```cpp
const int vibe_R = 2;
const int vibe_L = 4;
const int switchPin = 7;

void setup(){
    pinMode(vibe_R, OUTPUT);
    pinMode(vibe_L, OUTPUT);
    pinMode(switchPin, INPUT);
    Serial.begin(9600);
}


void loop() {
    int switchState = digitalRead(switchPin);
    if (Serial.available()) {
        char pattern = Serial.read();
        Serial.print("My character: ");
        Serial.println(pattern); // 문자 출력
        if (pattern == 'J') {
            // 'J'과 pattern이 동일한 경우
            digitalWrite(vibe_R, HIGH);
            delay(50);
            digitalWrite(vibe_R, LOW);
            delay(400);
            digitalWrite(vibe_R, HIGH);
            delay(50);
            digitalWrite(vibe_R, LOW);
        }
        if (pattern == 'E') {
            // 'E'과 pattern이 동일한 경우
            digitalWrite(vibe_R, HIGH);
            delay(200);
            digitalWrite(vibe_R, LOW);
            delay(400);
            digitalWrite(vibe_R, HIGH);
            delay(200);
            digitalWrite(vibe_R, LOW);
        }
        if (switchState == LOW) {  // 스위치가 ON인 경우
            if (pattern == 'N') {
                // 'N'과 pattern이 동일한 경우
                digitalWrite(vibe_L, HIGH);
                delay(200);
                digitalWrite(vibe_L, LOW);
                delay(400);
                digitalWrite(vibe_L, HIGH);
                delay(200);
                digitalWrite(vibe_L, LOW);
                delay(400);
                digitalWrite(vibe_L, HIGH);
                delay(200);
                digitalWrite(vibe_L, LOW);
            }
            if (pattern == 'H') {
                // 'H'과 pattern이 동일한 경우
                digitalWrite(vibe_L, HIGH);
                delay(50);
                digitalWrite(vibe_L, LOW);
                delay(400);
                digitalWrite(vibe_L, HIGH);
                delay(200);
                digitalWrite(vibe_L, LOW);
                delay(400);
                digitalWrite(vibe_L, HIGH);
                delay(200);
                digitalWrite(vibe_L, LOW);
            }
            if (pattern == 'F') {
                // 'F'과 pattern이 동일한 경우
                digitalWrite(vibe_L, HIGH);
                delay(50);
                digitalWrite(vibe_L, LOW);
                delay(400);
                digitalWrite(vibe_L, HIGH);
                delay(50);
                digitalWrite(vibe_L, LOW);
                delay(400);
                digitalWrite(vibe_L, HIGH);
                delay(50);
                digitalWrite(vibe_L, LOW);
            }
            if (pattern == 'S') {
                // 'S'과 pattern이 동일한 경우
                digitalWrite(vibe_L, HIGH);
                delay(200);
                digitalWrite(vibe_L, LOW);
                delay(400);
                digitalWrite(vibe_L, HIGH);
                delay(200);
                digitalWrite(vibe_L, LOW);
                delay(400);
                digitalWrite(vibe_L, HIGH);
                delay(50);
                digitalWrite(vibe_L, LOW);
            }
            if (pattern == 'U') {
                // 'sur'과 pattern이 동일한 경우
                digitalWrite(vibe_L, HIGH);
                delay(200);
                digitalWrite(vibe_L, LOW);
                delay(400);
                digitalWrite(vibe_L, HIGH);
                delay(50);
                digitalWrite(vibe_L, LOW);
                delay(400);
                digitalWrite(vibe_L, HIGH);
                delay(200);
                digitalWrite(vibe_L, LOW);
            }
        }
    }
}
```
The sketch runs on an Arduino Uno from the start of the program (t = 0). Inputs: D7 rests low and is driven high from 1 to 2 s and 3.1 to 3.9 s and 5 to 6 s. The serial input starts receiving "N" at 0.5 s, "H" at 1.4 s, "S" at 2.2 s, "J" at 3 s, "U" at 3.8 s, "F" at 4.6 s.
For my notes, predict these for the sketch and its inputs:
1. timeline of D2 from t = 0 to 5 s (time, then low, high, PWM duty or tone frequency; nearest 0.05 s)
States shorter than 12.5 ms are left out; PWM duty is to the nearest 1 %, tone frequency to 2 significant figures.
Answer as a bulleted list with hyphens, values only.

- 0 s low; 3.45 s high; 3.5 s low; 3.9 s high; 3.95 s low
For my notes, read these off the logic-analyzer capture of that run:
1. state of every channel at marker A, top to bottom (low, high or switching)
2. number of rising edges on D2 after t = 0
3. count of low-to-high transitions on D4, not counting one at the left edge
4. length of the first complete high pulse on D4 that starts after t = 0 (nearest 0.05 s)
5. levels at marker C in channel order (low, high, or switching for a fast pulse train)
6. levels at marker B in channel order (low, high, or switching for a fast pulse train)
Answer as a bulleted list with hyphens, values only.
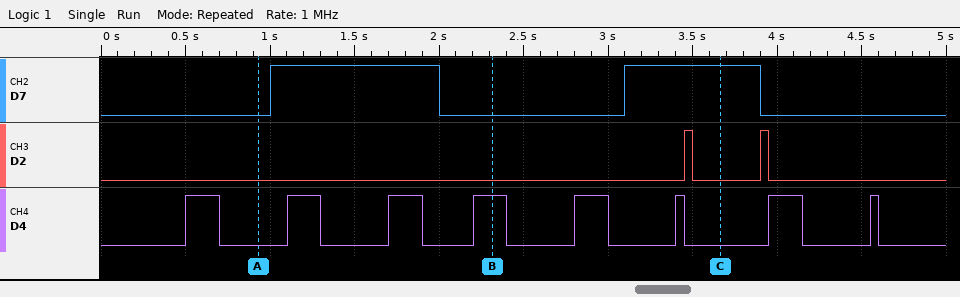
- D7 low, D2 low, D4 low
- 2
- 8
- 0.20 s
- D7 high, D2 low, D4 low
- D7 low, D2 low, D4 high
